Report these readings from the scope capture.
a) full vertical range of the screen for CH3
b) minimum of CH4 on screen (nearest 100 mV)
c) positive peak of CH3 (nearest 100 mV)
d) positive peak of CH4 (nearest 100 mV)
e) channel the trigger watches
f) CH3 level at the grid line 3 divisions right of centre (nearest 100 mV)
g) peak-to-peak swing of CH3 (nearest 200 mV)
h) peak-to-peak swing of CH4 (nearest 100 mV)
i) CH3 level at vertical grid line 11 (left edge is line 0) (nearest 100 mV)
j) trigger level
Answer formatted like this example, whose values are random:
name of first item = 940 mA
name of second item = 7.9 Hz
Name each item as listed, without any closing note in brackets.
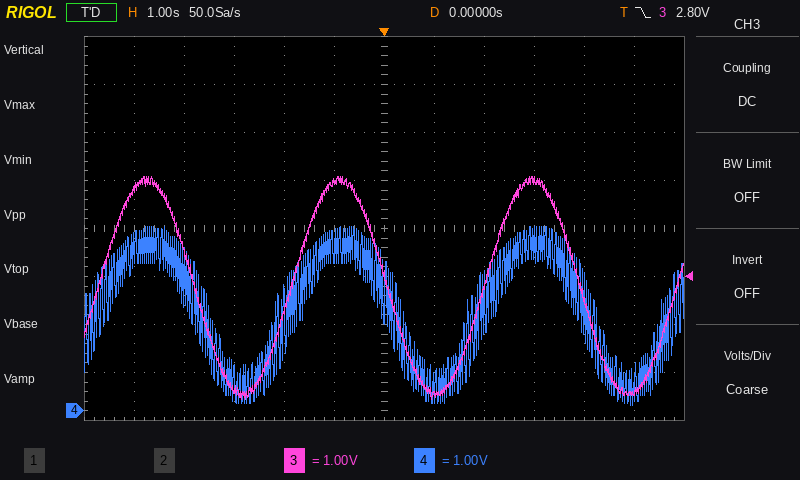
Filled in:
full vertical range of the screen for CH3 = 8 V
minimum of CH4 on screen = 100 mV
positive peak of CH3 = 4.9 V
positive peak of CH4 = 3.8 V
channel the trigger watches = CH3
CH3 level at the grid line 3 divisions right of centre = 4.8 V
peak-to-peak swing of CH3 = 4.6 V
peak-to-peak swing of CH4 = 3.7 V
CH3 level at vertical grid line 11 (left edge is line 0) = 400 mV
trigger level = 2.80 V
